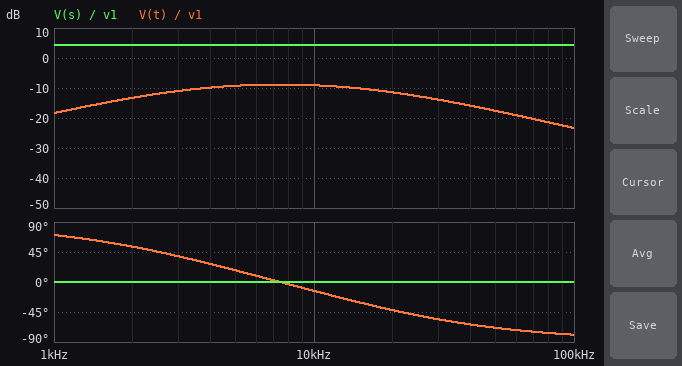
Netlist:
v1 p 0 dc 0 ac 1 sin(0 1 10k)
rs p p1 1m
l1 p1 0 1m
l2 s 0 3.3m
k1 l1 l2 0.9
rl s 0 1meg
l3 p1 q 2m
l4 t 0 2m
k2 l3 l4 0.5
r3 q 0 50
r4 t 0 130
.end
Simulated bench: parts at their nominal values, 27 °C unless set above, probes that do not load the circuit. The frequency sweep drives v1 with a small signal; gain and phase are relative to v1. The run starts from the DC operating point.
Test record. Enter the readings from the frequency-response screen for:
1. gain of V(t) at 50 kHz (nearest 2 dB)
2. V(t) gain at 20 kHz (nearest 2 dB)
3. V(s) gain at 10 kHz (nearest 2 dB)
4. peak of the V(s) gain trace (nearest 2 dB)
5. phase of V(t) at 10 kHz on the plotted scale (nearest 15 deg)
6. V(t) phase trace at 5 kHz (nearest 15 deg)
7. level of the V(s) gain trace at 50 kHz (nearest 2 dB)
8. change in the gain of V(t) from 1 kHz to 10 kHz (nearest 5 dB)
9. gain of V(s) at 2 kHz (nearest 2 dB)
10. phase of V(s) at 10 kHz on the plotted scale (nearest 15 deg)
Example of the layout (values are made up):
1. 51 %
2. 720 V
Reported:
1. -18 dB
2. -12 dB
3. 4 dB
4. 4 dB
5. -15 deg
6. 15 deg
7. 4 dB
8. 10 dB
9. 4 dB
10. 0 deg
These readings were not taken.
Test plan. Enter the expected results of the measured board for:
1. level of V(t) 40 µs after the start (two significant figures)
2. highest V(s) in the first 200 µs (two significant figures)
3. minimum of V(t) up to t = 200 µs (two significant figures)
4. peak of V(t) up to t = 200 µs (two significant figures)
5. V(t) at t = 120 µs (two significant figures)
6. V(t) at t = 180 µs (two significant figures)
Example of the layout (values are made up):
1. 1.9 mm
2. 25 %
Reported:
1. 200 mV
2. 1.6 V
3. -380 mV
4. 340 mV
5. 290 mV
6. -350 mV
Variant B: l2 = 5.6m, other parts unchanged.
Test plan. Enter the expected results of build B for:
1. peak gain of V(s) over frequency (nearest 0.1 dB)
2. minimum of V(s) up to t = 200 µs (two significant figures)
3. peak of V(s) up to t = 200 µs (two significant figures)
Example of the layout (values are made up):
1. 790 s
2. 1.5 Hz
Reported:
1. 6.6 dB
2. -2.1 V
3. 2.1 V
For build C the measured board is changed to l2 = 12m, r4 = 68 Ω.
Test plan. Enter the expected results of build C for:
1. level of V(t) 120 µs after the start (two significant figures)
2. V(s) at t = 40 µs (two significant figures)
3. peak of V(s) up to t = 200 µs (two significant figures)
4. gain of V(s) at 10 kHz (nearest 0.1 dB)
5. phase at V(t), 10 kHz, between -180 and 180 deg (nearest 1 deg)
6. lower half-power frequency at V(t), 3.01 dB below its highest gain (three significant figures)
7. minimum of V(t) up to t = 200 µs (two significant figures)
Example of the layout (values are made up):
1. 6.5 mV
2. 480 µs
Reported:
1. 150 mV
2. 1.8 V
3. 3.1 V
4. 9.9 dB
5. -30 deg
6. 1.98 kHz
7. -280 mV
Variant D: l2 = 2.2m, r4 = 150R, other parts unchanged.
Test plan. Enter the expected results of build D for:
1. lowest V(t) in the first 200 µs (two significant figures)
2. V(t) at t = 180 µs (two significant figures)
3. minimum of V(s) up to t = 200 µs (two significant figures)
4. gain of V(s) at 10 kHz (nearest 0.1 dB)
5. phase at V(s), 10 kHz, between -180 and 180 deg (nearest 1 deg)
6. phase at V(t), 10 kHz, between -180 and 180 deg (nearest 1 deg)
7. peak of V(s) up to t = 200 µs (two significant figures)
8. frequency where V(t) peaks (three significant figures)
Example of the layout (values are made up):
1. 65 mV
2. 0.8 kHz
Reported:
1. -400 mV
2. -370 mV
3. -1.3 V
4. 2.5 dB
5. 0 deg
6. -10 deg
7. 1.3 V
8. 7.96 kHz
